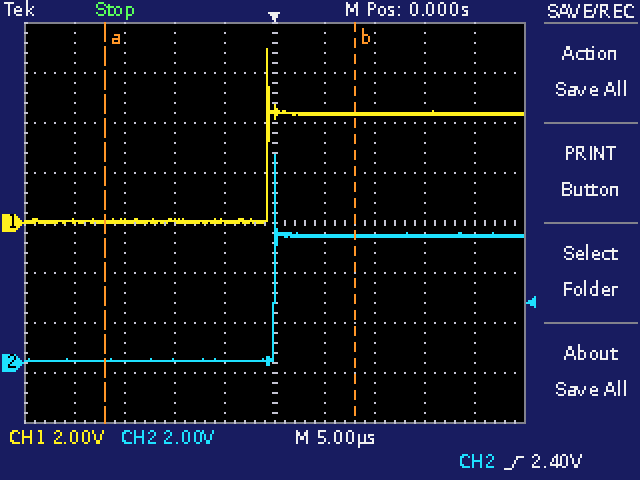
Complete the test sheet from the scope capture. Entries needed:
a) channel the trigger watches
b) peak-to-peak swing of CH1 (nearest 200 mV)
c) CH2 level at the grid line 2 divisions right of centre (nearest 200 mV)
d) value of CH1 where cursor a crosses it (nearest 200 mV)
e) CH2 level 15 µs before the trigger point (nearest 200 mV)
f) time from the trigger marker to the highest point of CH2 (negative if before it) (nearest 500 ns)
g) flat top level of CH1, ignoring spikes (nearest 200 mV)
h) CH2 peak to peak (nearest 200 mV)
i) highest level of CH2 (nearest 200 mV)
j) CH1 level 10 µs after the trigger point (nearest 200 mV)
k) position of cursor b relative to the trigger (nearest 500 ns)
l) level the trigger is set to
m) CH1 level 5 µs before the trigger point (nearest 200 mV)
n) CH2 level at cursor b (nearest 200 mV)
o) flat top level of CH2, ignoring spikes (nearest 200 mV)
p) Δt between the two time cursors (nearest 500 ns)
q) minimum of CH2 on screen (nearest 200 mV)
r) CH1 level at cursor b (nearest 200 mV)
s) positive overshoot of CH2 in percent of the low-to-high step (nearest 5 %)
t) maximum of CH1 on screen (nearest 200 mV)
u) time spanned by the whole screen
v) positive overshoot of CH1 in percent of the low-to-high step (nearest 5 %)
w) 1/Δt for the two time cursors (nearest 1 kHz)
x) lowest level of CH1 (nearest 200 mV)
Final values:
CH2
7.0 V
5.0 V
0.0 V
0.0 V
0.0 µs
4.4 V
8.4 V
8.4 V
4.4 V
+8.0 µs
2.40 V
0.0 V
5.0 V
5.0 V
25.0 µs
0.0 V
4.4 V
65 %
7.0 V
50 µs
60 %
40 kHz
0.0 V
